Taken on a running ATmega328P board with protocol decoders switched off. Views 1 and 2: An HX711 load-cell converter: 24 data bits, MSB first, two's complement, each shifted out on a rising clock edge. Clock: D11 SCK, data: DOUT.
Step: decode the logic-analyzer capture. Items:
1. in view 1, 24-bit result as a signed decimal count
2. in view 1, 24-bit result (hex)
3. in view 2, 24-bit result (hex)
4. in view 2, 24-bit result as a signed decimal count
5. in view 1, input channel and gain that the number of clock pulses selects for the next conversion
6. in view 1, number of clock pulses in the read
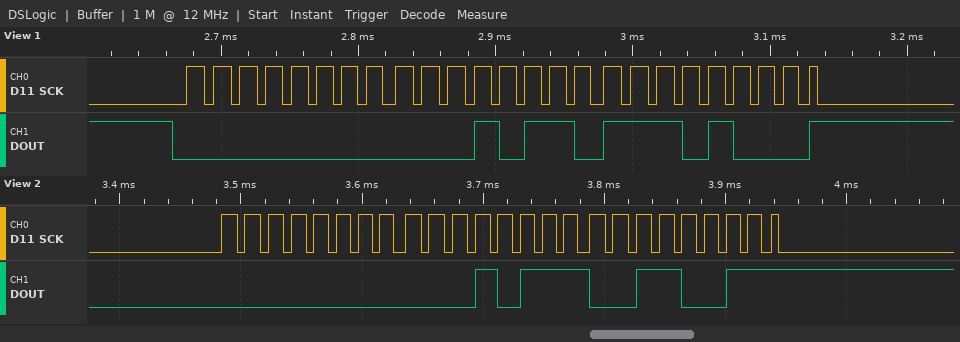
5864
0x0016E8
0x001733
5939
channel A, gain 128
25
